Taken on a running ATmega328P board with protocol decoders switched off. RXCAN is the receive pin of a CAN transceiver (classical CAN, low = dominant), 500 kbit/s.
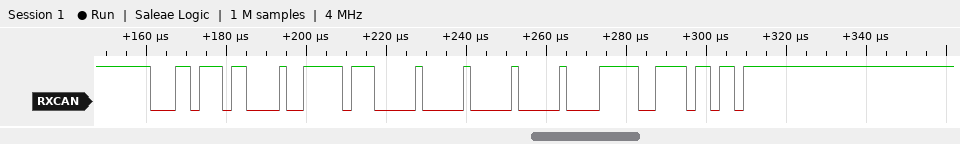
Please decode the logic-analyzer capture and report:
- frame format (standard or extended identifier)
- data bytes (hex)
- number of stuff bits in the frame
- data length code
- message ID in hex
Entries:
standard
FF 00 00 00
6
4
0x1BB
